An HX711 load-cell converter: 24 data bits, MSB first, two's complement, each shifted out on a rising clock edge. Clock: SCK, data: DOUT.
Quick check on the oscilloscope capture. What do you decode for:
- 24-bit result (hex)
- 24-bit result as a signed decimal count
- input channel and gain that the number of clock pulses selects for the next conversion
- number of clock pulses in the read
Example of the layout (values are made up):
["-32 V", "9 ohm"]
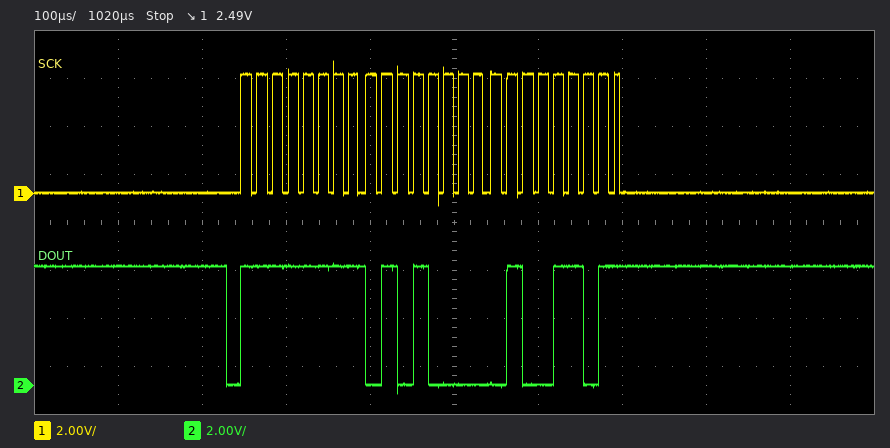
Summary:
["0xFF504D", "-44979", "channel A, gain 128", "25"]
